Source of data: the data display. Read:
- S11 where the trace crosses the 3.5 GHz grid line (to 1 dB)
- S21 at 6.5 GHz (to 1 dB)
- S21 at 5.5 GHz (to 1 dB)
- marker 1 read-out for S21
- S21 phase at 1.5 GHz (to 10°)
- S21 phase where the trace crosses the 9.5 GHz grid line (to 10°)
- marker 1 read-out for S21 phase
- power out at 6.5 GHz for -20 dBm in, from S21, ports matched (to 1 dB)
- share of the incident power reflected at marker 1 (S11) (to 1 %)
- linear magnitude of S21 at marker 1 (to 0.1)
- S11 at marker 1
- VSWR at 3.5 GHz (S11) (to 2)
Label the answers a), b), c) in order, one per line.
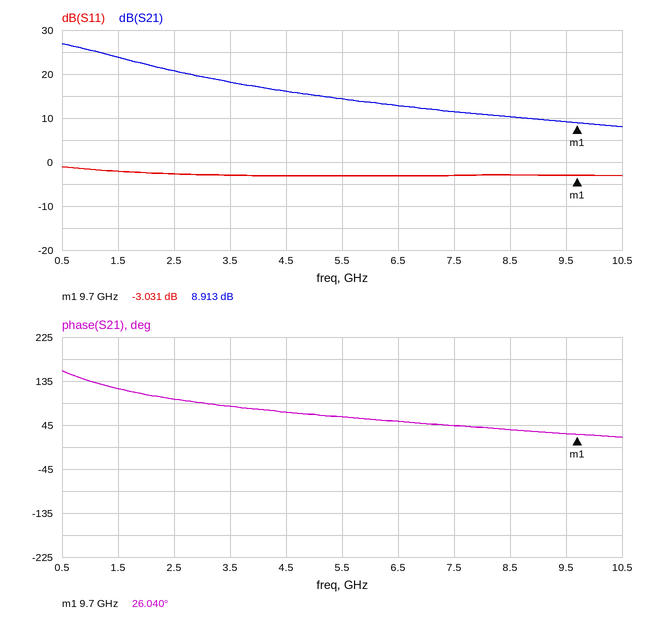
a) -3 dB
b) 13 dB
c) 14 dB
d) 8.913 dB
e) 120°
f) 30°
g) 26.040°
h) -7 dBm
i) 50 %
j) 2.8
k) -3.031 dB
l) 6
